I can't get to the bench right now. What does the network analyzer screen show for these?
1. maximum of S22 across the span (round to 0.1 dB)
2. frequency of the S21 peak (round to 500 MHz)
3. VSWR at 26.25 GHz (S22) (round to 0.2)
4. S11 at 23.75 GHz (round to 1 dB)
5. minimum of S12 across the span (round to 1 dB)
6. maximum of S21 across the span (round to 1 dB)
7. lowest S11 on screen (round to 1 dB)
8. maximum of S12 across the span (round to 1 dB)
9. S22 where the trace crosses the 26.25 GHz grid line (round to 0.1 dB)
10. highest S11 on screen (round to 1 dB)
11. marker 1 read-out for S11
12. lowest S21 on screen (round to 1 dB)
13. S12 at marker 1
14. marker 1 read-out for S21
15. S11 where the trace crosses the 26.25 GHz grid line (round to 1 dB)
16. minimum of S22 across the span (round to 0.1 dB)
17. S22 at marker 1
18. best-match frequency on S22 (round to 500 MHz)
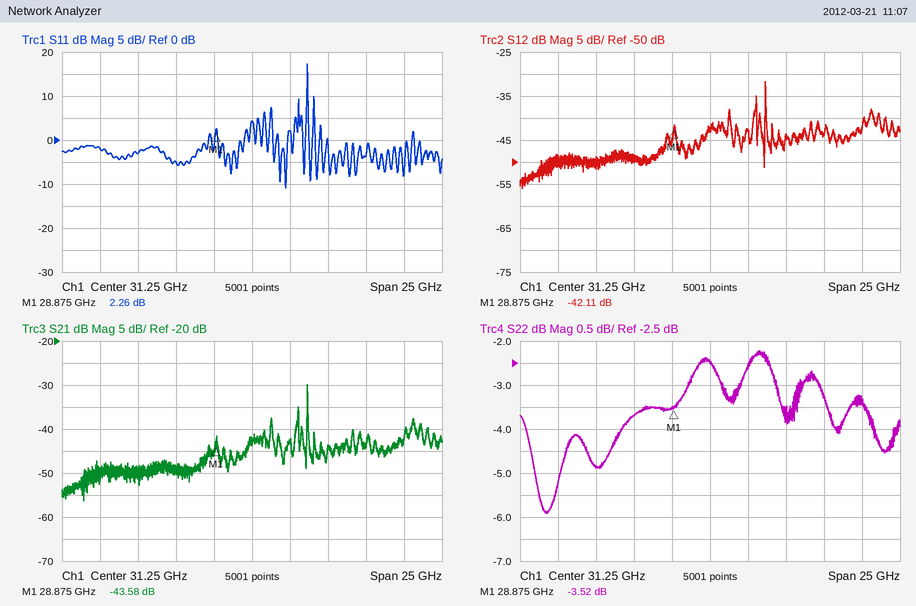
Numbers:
-2.2 dB
35.0 GHz
4.8
-3 dB
-56 dB
-30 dB
-11 dB
-32 dB
-3.7 dB
17 dB
2.26 dB
-56 dB
-42.11 dB
-43.58 dB
-5 dB
-5.9 dB
-3.52 dB
20.5 GHz
